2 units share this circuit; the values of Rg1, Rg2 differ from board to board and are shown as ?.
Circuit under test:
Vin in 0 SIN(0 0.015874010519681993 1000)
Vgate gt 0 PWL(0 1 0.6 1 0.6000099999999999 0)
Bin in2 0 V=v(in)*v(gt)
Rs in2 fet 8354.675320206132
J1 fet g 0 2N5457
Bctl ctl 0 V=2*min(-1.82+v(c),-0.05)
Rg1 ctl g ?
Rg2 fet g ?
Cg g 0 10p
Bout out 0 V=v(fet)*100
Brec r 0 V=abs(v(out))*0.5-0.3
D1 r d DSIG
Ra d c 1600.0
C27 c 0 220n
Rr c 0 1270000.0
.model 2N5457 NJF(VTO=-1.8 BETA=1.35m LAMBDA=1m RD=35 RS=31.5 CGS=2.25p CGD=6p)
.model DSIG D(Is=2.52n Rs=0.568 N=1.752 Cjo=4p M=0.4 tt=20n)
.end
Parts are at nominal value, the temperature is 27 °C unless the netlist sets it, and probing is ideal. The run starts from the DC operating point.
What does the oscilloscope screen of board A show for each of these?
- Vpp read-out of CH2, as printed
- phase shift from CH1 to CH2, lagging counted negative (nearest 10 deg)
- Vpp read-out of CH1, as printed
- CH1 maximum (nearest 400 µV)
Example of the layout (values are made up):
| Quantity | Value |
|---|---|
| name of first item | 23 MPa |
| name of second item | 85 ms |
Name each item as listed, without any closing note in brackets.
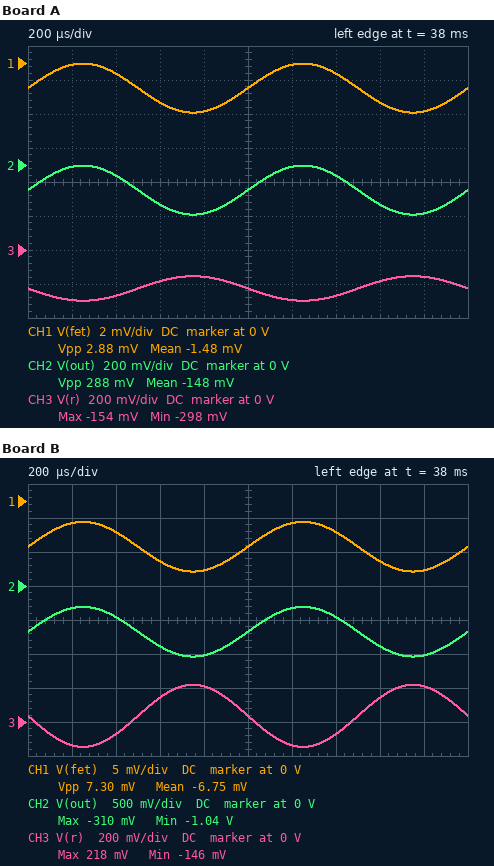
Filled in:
| Quantity | Value |
|---|---|
| Vpp read-out of CH2, as printed | 288 mV |
| phase shift from CH1 to CH2, lagging counted negative | 0 deg |
| Vpp read-out of CH1, as printed | 2.88 mV |
| CH1 maximum | 0 V |
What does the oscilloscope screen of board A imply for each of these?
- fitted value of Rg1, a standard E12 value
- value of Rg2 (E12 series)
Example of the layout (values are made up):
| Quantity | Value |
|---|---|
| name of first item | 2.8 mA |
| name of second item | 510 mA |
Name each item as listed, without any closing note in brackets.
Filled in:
| Quantity | Value |
|---|---|
| fitted value of Rg1, a standard E12 value | 1.2 MΩ |
| value of Rg2 | 680 kΩ |
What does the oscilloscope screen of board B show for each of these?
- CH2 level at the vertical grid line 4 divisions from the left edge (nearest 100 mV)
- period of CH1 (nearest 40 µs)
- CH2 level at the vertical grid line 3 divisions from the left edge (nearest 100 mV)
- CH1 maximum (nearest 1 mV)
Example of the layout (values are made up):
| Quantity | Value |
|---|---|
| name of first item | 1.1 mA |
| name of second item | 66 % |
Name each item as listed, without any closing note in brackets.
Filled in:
| Quantity | Value |
|---|---|
| CH2 level at the vertical grid line 4 divisions from the left edge | -1.0 V |
| period of CH1 | 1.00 ms |
| CH2 level at the vertical grid line 3 divisions from the left edge | -900 mV |
| CH1 maximum | -3 mV |
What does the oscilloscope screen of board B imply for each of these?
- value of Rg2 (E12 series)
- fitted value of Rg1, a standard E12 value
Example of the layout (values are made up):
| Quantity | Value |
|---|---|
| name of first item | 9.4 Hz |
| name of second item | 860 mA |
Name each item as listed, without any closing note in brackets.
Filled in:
| Quantity | Value |
|---|---|
| value of Rg2 | 470 kΩ |
| fitted value of Rg1, a standard E12 value | 560 kΩ |
